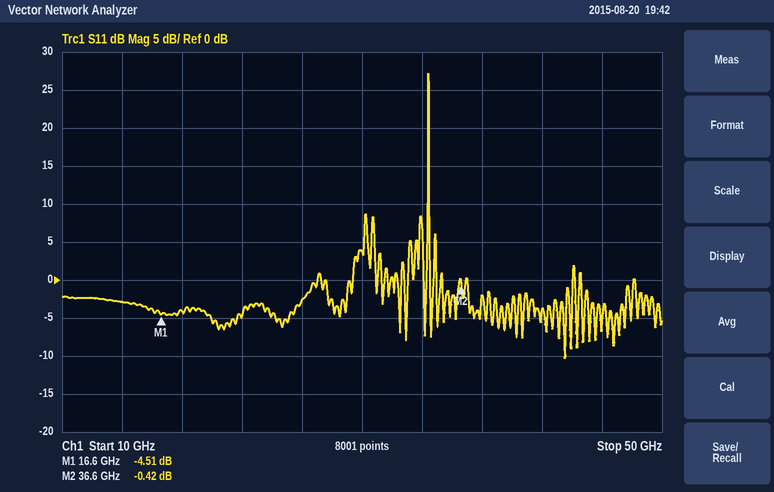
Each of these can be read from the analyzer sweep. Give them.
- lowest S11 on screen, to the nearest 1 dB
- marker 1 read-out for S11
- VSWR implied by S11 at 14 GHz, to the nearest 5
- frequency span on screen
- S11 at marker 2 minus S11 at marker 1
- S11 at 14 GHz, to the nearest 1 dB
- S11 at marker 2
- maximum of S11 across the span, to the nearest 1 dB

-10 dB
-4.51 dB
5
40 GHz
4.09 dB
-3 dB
-0.42 dB
27 dB
